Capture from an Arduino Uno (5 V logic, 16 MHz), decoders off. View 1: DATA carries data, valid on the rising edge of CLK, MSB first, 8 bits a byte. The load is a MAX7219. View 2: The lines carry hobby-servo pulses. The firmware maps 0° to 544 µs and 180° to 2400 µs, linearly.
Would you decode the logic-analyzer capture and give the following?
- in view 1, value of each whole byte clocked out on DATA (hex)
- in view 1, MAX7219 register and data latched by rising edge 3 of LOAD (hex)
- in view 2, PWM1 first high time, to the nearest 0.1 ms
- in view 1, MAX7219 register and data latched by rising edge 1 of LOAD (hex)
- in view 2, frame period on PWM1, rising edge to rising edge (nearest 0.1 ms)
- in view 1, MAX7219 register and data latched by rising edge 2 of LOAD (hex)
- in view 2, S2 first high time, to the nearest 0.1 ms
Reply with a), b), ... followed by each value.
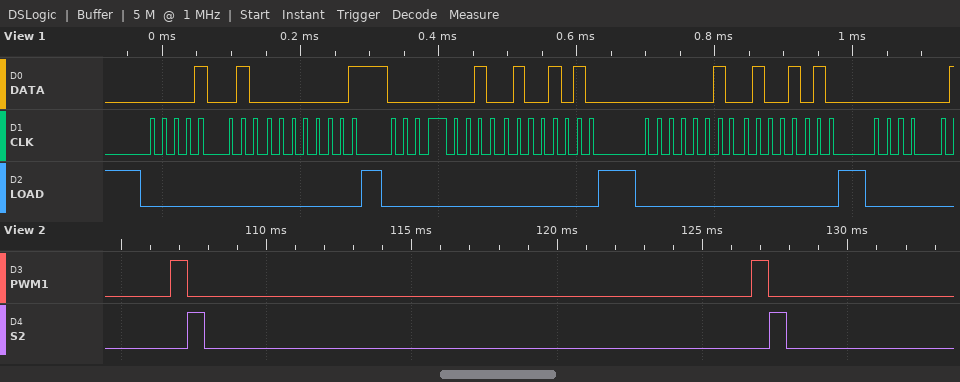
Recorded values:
a) 0A 01 02 4A 02 4A
b) register 0x2, data 0x4A
c) 0.6 ms
d) register 0xA, data 0x01
e) 20.0 ms
f) register 0x2, data 0x4A
g) 0.6 ms
